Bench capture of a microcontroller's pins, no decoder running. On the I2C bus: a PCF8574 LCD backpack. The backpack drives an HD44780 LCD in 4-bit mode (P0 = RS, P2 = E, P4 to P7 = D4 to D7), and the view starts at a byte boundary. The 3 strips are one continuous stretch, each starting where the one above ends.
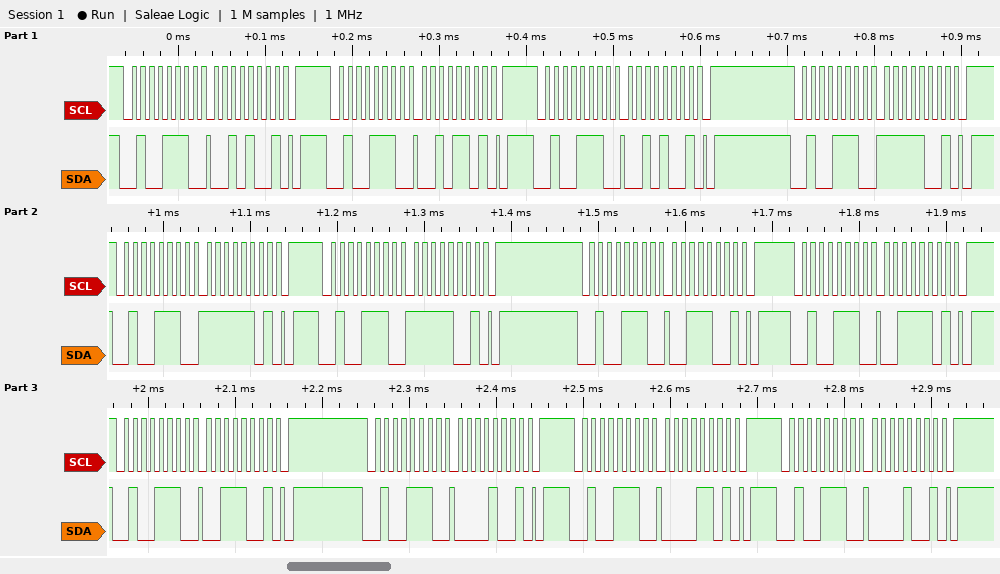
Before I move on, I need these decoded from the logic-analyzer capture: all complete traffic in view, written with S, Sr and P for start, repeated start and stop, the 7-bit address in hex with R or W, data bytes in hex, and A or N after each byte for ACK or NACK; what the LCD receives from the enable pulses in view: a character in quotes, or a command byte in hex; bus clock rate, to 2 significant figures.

S 27W A 29 A P S 27W A 2D A P S 27W A 29 A P S 27W A F9 A P S 27W A FD A P S 27W A F9 A P S 27W A 39 A P S 27W A 3D A P S 27W A 39 A P S 27W A 09 A P S 27W A 0D A P S 27W A 09 A P
'/' '0'
100 kHz
